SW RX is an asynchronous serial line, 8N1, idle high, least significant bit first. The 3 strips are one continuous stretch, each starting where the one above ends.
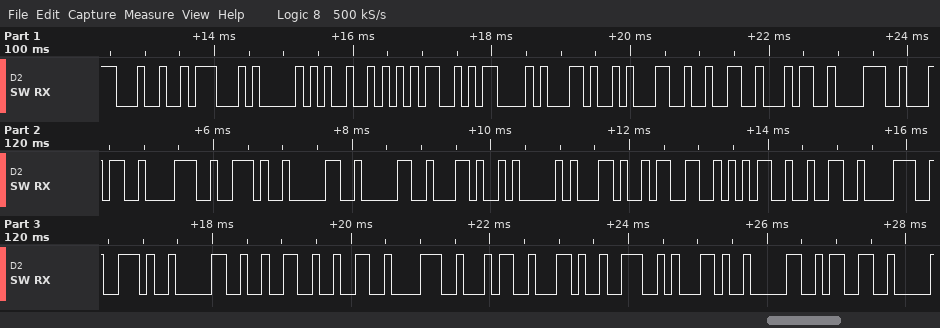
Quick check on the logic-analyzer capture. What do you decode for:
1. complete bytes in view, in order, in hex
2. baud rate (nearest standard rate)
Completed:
24 47 50 52 4D 43 2C 31 32 34 38 34 38 2E 30 30 2C 41 2C 33 35 32 38 2E 30 32 32 38 34 2C 4E 2C 30 33
9600 baud
